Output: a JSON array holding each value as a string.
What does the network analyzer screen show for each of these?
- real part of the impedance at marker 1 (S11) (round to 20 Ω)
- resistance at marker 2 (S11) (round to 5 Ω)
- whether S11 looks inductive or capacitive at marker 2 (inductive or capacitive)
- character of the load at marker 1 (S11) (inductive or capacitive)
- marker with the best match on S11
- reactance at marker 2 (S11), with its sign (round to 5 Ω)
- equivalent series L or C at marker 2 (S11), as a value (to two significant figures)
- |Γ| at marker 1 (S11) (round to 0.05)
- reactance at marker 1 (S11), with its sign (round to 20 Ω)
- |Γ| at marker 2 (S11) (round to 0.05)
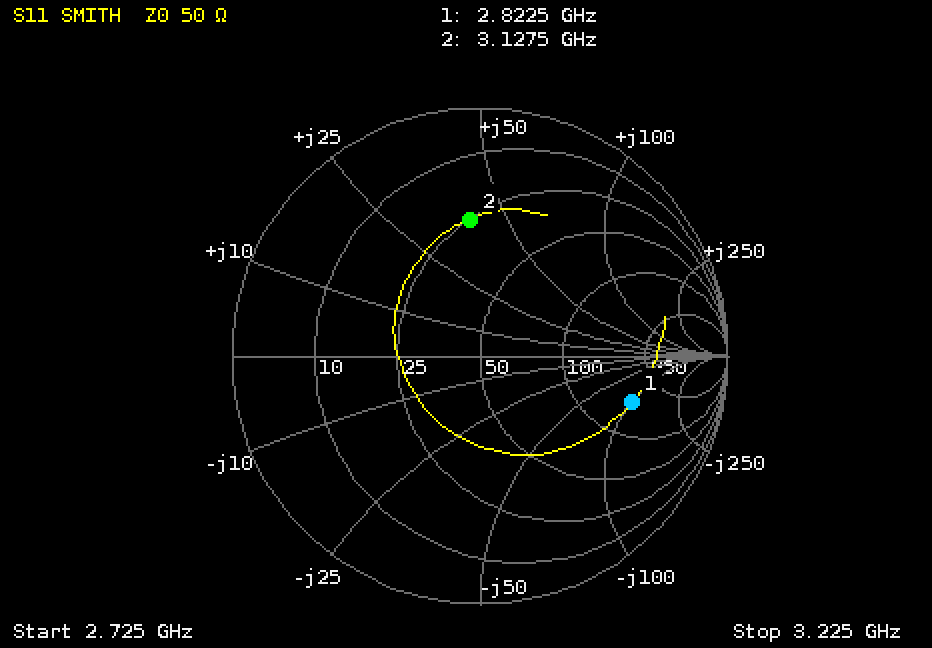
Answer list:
["160 Ω", "25 Ω", "inductive", "capacitive", "marker 2", "+40 Ω", "2.0 nH", "0.65", "-100 Ω", "0.55"]
